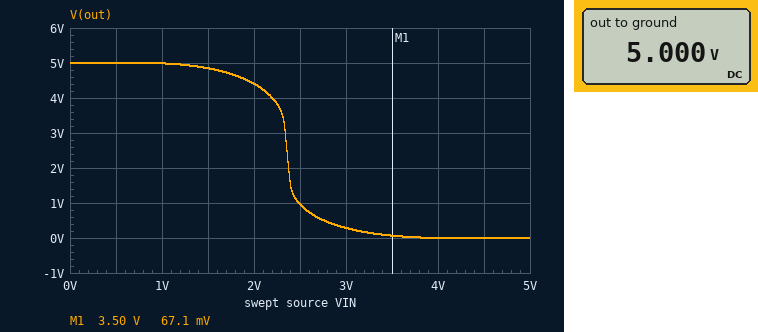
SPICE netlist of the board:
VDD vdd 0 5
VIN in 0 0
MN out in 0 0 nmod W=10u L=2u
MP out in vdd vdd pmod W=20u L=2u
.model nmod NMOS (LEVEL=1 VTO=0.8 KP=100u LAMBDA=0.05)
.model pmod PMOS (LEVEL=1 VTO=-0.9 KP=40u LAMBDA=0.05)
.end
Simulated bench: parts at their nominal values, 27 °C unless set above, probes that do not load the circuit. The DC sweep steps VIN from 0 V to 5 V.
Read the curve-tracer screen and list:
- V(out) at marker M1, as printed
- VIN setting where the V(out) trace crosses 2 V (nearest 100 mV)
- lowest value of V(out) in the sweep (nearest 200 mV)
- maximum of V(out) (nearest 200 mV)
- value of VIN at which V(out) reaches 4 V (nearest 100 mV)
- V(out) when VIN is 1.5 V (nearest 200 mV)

67.1 mV
2.4 V
0 V
5.0 V
2.2 V
4.8 V
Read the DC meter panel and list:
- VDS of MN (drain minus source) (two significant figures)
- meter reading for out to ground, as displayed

5.0 V
5.000 V
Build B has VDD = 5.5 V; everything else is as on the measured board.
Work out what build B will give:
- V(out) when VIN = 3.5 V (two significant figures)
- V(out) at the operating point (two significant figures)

230 mV
5.5 V
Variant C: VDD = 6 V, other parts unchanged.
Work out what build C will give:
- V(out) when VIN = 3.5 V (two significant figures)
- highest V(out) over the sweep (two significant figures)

520 mV
6.0 V
